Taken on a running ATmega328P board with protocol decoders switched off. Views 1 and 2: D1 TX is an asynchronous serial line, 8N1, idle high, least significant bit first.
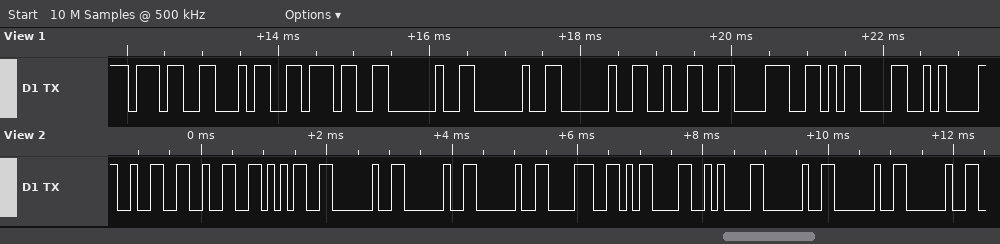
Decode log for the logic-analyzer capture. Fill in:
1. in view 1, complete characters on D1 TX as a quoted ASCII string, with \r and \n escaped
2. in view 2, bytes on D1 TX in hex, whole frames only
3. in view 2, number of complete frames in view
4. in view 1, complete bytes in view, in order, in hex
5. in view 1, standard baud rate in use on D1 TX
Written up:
"747   28\r\n"
32 32 35 20 20 20 38 0D 0A 20 20 20
12
37 34 37 20 20 20 32 38 0D 0A
9600 baud
